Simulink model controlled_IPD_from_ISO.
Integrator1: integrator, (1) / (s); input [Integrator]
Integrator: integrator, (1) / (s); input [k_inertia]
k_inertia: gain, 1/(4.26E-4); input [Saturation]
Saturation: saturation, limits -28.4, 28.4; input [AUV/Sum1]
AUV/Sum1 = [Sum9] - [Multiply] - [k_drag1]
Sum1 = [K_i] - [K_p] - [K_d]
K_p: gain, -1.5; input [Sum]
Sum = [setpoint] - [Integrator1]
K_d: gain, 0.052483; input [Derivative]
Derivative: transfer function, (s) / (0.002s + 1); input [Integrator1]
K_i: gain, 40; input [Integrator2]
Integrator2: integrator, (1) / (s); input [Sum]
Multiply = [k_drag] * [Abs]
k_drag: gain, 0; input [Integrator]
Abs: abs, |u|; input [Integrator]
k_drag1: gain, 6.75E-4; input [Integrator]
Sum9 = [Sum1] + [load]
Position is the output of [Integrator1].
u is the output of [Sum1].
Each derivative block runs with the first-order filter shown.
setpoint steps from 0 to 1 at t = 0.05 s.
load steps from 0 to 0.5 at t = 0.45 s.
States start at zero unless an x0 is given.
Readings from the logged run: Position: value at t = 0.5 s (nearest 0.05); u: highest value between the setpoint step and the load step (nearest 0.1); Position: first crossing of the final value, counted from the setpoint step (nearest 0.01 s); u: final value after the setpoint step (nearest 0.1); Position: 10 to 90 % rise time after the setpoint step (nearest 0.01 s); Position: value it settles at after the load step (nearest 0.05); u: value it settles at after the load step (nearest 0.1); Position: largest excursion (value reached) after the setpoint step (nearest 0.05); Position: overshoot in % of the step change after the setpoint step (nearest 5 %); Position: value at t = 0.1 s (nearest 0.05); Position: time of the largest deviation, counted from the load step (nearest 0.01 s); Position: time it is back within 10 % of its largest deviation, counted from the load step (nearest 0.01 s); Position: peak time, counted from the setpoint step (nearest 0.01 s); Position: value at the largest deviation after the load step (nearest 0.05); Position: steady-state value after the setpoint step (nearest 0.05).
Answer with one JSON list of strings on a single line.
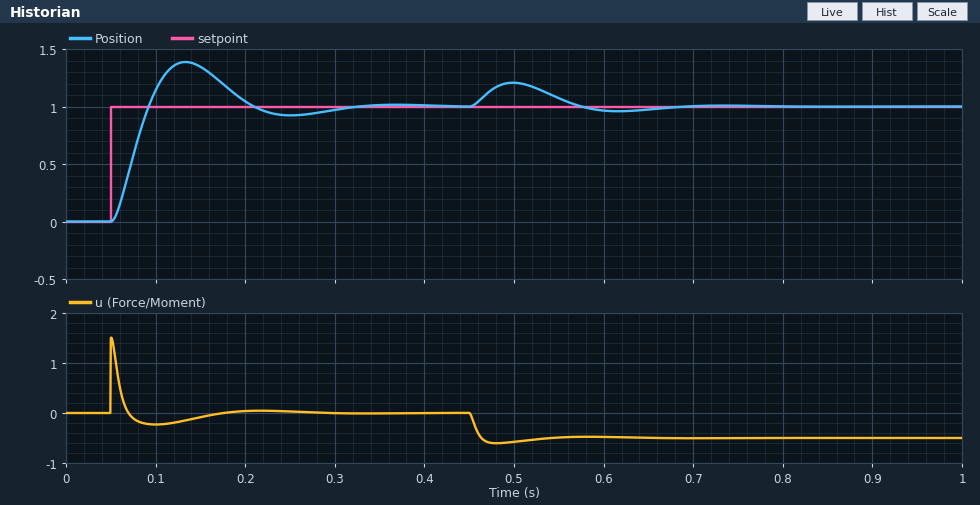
["1.20", "1.5", "0.04 s", "0.0", "0.03 s", "1.00", "-0.5", "1.40", "40 %", "1.15", "0.05 s", "0.21 s", "0.08 s", "1.20", "1.00"]
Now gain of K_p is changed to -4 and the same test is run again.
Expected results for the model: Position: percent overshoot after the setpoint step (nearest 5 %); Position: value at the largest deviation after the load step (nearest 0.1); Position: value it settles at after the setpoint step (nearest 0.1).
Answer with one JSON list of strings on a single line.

["15 %", "1.1", "1.0"]
